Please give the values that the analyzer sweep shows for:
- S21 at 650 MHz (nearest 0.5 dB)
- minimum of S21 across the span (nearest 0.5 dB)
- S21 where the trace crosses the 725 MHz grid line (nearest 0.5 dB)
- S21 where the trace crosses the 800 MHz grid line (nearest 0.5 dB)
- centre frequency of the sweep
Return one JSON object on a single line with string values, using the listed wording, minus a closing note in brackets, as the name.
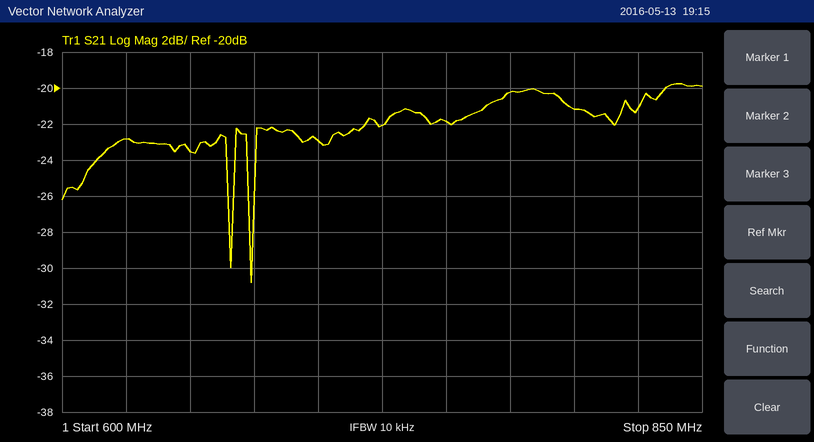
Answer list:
{"S21 at 650 MHz": "-23.5 dB", "minimum of S21 across the span": "-31.0 dB", "S21 where the trace crosses the 725 MHz grid line": "-22.0 dB", "S21 where the trace crosses the 800 MHz grid line": "-21.0 dB", "centre frequency of the sweep": "725 MHz"}
